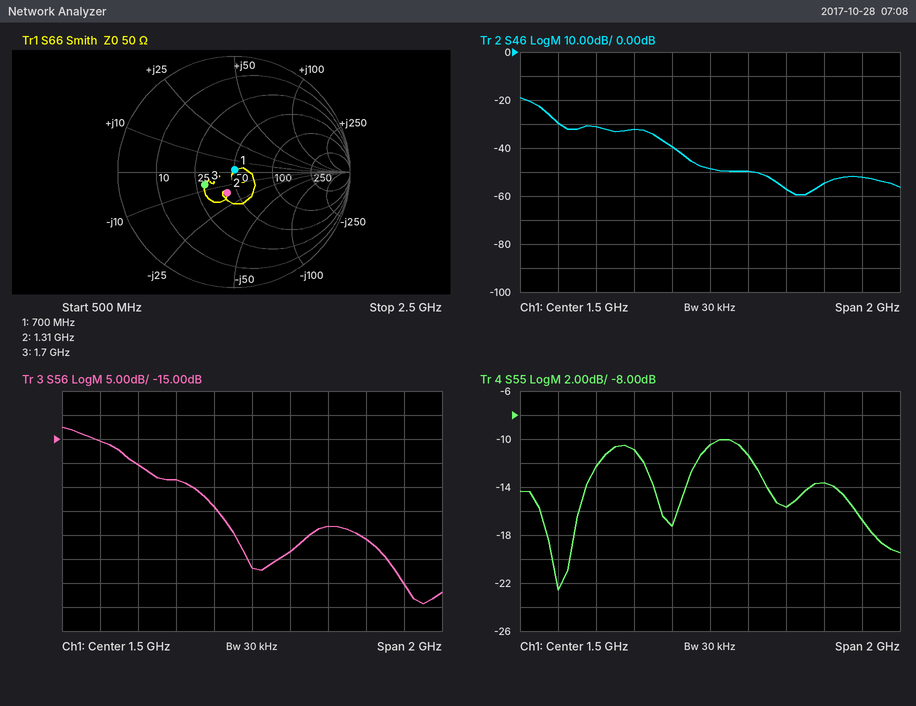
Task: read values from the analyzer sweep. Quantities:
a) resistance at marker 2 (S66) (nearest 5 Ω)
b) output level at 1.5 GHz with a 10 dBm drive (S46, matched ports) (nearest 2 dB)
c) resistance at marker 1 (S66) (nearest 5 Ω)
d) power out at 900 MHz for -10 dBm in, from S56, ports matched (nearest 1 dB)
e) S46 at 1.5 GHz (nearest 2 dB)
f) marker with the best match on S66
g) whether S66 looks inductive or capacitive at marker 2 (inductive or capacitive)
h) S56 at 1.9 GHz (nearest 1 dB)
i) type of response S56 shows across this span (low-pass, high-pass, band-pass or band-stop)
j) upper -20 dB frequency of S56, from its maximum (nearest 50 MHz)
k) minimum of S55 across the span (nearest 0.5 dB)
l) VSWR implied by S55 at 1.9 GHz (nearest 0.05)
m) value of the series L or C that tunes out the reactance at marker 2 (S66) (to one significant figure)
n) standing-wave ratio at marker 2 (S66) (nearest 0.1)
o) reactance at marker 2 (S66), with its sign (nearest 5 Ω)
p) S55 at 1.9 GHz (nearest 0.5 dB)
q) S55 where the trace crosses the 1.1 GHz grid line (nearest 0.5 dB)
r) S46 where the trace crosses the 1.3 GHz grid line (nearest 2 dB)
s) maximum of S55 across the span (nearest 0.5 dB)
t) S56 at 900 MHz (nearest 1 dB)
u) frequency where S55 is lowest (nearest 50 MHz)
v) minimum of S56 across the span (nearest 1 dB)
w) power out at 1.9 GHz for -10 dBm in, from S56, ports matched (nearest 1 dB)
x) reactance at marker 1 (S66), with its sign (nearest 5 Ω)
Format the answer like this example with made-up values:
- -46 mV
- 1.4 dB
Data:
- 40 Ω
- -38 dBm
- 50 Ω
- -30 dBm
- -48 dB
- marker 1
- capacitive
- -33 dB
- low-pass
- 1.35 GHz
- -22.5 dB
- 1.40
- 2 nH
- 1.5
- -15 Ω
- -15.5 dB
- -11.0 dB
- -40 dB
- -10.0 dB
- -20 dB
- 700 MHz
- -49 dB
- -43 dBm
- 0 Ω
